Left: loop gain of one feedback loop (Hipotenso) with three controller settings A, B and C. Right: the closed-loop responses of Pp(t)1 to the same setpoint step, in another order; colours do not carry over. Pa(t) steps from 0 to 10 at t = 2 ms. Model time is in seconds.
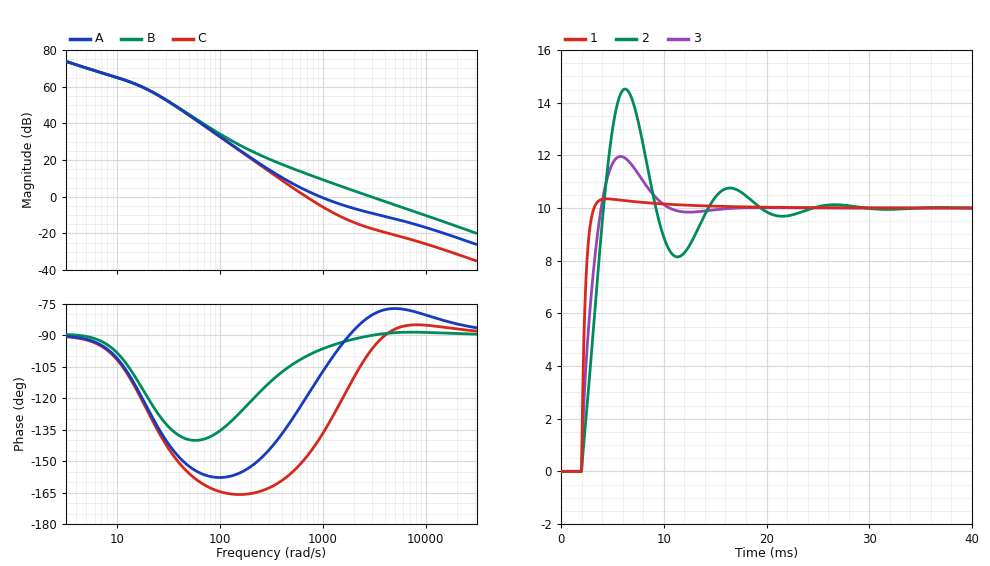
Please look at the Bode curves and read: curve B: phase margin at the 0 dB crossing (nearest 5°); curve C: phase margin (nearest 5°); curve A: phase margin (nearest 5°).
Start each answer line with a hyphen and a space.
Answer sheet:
- 90°
- 30°
- 70°
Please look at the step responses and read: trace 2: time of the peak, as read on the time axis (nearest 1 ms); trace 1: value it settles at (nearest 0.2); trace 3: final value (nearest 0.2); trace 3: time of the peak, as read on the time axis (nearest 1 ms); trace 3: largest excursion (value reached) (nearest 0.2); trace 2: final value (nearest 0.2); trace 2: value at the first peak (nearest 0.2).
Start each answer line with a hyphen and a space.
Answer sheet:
- 6 ms
- 10.0
- 10.0
- 6 ms
- 12.0
- 10.0
- 14.6
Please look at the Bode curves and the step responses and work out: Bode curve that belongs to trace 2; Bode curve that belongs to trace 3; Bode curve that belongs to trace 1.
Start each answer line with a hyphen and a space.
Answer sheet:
- C
- A
- B
